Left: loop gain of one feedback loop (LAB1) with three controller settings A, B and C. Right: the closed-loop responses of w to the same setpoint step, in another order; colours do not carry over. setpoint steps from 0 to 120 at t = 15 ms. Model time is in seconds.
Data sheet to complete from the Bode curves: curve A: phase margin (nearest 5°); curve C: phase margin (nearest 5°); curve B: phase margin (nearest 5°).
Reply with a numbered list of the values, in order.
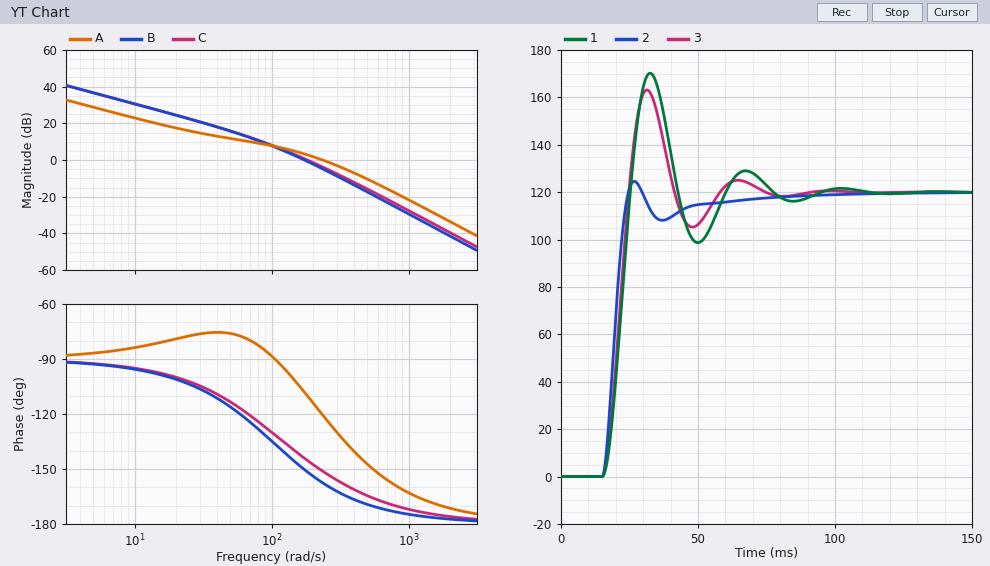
1. 60°
2. 35°
3. 30°
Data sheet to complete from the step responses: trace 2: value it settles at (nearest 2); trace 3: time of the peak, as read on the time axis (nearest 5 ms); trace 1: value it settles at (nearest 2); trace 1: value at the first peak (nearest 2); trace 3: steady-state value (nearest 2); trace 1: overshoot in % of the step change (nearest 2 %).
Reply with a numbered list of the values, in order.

1. 120
2. 30 ms
3. 120
4. 170
5. 120
6. 42 %
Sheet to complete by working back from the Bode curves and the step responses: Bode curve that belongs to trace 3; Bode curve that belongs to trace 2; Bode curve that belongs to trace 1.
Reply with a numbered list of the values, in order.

1. C
2. A
3. B
